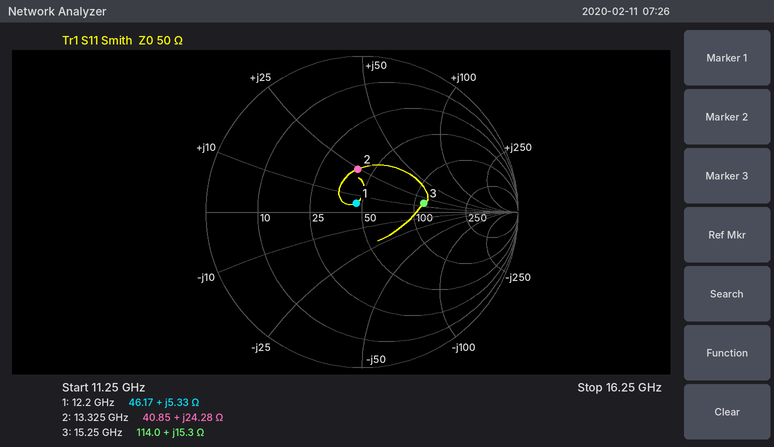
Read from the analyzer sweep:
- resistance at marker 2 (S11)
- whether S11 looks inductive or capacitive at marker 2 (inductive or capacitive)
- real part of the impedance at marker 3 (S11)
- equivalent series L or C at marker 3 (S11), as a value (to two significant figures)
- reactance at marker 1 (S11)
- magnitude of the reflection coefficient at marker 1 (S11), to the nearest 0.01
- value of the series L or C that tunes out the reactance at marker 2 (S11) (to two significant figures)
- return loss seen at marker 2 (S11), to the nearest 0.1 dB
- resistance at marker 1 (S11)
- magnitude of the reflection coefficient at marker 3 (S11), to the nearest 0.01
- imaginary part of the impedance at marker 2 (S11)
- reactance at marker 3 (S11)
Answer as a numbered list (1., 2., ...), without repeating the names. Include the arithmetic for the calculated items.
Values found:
1. 40.85 Ω
2. inductive
3. 114.0 Ω
4. L = 15.3 Ω/(2π × 15.25 GHz) ≈ 160 pH
5. +5.33 Ω
6. 0.07
7. C = 1/(2π × 13.325 GHz × 24.28 Ω) ≈ 492 fF, so 490 fF to two significant figures
8. 11.2 dB
9. 46.17 Ω
10. 0.40
11. +24.28 Ω
12. +15.3 Ω
